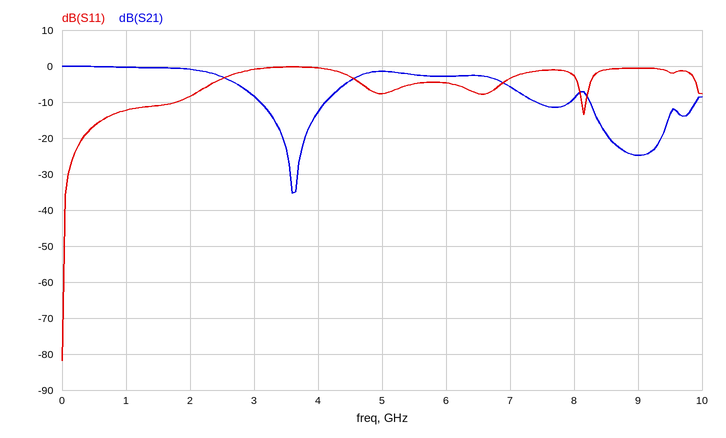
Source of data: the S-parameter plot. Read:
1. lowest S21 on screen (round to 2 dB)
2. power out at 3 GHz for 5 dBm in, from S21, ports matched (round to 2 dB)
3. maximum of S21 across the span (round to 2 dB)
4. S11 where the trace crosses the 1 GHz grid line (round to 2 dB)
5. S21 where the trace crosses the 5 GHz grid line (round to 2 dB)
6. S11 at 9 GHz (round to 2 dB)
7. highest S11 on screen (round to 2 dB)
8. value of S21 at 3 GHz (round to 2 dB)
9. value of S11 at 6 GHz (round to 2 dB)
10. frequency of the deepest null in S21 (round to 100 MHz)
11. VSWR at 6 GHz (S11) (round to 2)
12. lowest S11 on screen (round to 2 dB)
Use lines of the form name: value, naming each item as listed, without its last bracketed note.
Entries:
lowest S21 on screen: -36 dB
power out at 3 GHz for 5 dBm in, from S21, ports matched: -4 dBm
maximum of S21 across the span: 0 dB
S11 where the trace crosses the 1 GHz grid line: -12 dB
S21 where the trace crosses the 5 GHz grid line: -2 dB
S11 at 9 GHz: 0 dB
highest S11 on screen: 0 dB
value of S21 at 3 GHz: -8 dB
value of S11 at 6 GHz: -4 dB
frequency of the deepest null in S21: 3.6 GHz
VSWR at 6 GHz (S11): 4
lowest S11 on screen: -82 dB
